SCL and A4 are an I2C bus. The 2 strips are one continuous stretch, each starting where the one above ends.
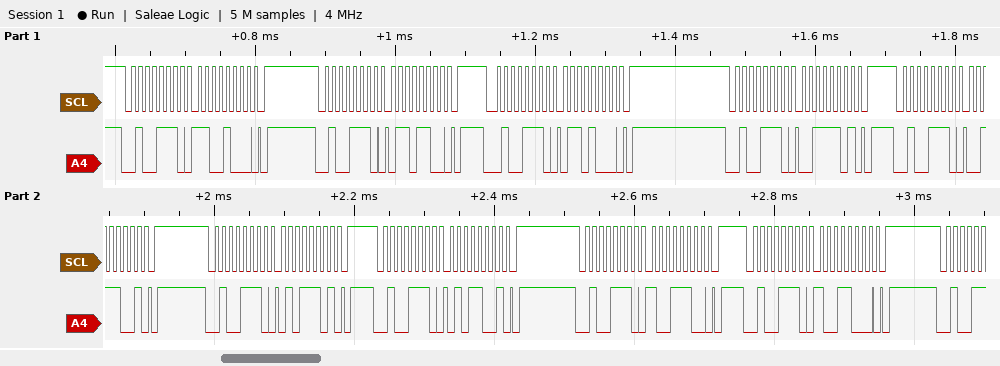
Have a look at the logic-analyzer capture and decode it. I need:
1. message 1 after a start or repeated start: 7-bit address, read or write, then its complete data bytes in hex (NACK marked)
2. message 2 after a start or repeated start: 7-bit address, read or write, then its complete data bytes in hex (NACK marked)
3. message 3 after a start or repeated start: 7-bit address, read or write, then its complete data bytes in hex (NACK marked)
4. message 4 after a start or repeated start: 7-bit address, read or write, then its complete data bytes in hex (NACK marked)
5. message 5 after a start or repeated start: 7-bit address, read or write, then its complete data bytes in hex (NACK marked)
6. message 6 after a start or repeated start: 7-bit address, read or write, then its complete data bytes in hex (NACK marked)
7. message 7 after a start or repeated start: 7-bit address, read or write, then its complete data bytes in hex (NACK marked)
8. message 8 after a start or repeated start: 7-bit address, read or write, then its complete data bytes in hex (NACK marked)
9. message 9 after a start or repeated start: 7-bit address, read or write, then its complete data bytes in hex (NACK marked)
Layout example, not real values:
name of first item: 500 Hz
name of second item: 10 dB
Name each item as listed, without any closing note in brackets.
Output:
message 1 after a start or repeated start: 7-bit address, read or write, then its complete data bytes in hex: 0x27 write: C8
message 2 after a start or repeated start: 7-bit address, read or write, then its complete data bytes in hex: 0x27 write: 6C
message 3 after a start or repeated start: 7-bit address, read or write, then its complete data bytes in hex: 0x27 write: 68
message 4 after a start or repeated start: 7-bit address, read or write, then its complete data bytes in hex: 0x27 write: 3D
message 5 after a start or repeated start: 7-bit address, read or write, then its complete data bytes in hex: 0x27 write: 39
message 6 after a start or repeated start: 7-bit address, read or write, then its complete data bytes in hex: 0x27 write: 5D
message 7 after a start or repeated start: 7-bit address, read or write, then its complete data bytes in hex: 0x27 write: 59
message 8 after a start or repeated start: 7-bit address, read or write, then its complete data bytes in hex: 0x27 write: 9C
message 9 after a start or repeated start: 7-bit address, read or write, then its complete data bytes in hex: 0x27 write: 98
